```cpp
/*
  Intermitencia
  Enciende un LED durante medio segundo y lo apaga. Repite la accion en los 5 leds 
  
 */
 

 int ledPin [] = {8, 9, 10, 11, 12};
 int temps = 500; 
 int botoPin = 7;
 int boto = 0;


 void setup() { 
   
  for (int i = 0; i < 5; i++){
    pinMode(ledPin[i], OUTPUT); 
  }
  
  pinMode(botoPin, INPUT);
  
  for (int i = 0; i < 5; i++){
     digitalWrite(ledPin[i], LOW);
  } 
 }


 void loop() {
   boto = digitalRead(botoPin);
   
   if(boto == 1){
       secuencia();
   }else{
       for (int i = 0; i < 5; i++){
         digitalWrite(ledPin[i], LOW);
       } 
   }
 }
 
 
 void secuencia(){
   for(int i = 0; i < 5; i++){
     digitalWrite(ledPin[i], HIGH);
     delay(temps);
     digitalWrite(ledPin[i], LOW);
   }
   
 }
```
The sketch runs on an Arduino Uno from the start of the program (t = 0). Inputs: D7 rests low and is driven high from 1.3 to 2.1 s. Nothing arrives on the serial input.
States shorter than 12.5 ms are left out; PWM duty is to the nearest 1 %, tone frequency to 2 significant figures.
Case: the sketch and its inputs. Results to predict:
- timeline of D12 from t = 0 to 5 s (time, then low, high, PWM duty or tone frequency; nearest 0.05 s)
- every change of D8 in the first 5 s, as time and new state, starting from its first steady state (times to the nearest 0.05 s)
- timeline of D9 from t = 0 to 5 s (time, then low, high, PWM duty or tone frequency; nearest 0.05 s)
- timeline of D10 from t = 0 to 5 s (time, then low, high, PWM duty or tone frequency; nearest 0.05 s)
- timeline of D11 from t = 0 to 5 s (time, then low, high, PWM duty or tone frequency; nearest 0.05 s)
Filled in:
0 s low; 3.3 s high; 3.8 s low
0 s low; 1.3 s high; 1.8 s low
0 s low; 1.8 s high; 2.3 s low
0 s low; 2.3 s high; 2.8 s low
0 s low; 2.8 s high; 3.3 s low
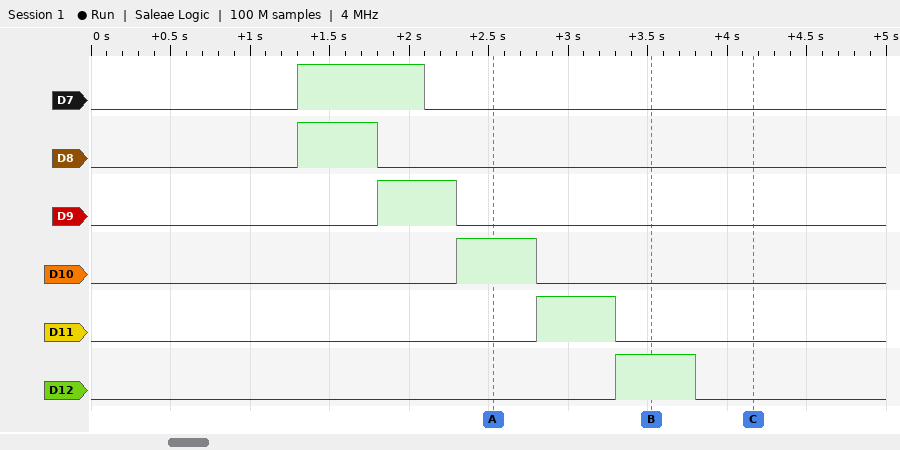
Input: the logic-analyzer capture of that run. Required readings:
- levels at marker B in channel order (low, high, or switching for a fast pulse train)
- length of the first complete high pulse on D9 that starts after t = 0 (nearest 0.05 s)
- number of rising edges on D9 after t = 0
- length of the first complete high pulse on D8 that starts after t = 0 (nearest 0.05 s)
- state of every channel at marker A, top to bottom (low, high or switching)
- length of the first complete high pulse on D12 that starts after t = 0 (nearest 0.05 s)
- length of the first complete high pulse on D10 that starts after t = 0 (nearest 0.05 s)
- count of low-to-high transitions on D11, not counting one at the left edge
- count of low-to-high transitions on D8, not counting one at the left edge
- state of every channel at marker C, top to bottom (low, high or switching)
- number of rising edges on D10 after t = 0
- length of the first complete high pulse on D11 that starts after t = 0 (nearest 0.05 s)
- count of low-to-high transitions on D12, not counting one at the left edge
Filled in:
D7 low, D8 low, D9 low, D10 low, D11 low, D12 high
0.50 s
1
0.50 s
D7 low, D8 low, D9 low, D10 high, D11 low, D12 low
0.50 s
0.50 s
1
1
D7 low, D8 low, D9 low, D10 low, D11 low, D12 low
1
0.50 s
1
